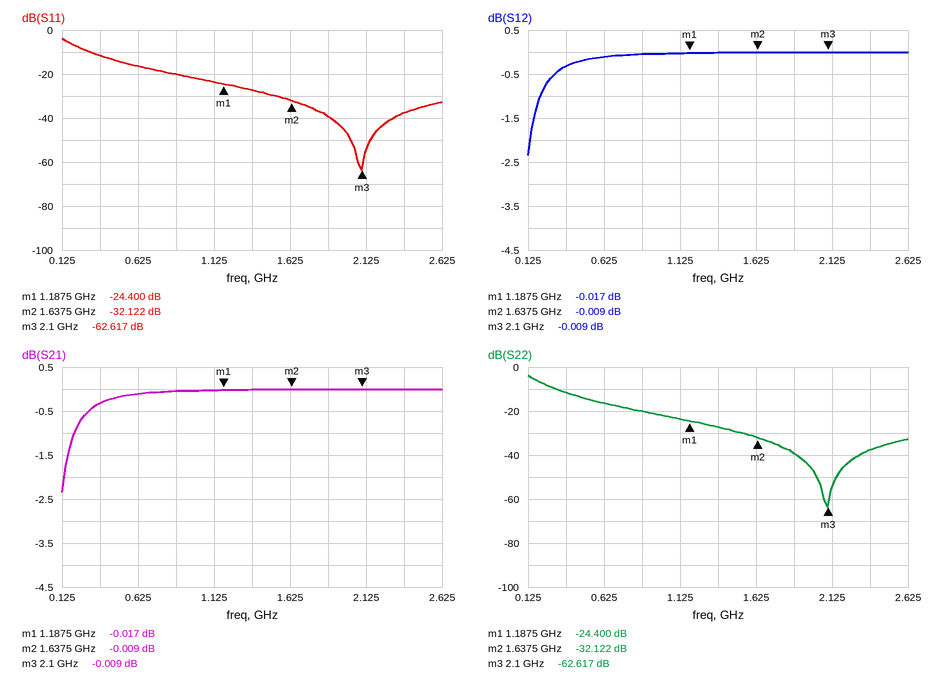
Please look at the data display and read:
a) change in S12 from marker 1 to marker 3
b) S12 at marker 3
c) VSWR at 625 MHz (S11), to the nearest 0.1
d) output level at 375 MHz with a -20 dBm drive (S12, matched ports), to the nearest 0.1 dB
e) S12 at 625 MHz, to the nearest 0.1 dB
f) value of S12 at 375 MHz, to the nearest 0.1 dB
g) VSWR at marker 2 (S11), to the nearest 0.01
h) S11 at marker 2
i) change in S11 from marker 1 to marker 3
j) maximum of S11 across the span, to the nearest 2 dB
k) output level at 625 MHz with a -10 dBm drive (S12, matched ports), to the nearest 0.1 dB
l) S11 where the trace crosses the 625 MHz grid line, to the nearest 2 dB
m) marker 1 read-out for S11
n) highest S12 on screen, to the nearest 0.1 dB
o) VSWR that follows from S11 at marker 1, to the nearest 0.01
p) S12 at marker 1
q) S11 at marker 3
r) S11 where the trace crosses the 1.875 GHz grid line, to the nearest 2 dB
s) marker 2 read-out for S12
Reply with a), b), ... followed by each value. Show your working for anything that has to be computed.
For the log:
a) -0.009 − (-0.017) = 0.008 dB
b) -0.009 dB
c) |Γ| = 10^(-16/20) = 0.1585; VSWR = (1 + 0.1585)/(1 − 0.1585) ≈ 1.4
d) -20 dBm + (-0.3 dB) = -20.3 dBm
e) -0.1 dB
f) -0.3 dB
g) (1 + 0.0248)/(1 − 0.0248) ≈ 1.05
h) -32.122 dB
i) -62.617 − (-24.4) = -38.217 dB
j) -4 dB
k) -10 dBm + (-0.1 dB) = -10.1 dBm
l) -16 dB
m) -24.400 dB
n) 0.0 dB
o) (1 + 0.0603)/(1 − 0.0603) ≈ 1.13
p) -0.017 dB
q) -62.617 dB
r) -40 dB
s) -0.009 dB
